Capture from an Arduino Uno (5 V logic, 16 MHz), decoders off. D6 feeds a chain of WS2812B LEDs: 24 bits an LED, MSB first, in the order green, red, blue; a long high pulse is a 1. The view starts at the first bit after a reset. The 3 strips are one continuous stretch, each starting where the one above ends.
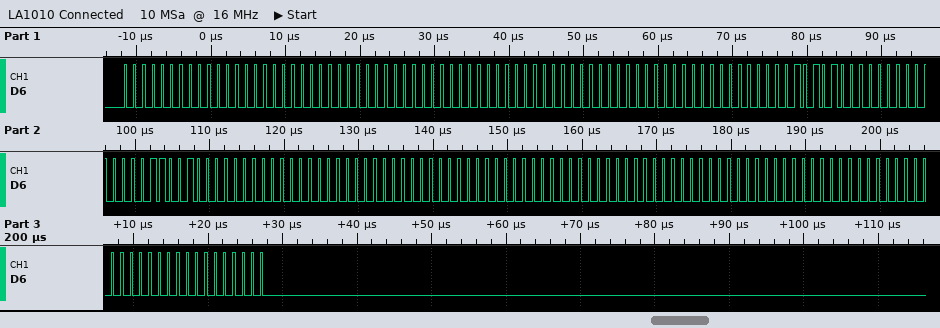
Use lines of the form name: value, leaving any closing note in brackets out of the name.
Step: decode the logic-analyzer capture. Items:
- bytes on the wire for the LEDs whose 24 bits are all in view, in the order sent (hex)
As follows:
bytes on the wire for the LEDs whose 24 bits are all in view, in the order sent: 00 00 00 00 00 00 00 00 00 A8 00 19 00 00 00 00 00 00 00 00 00 00 00 00
